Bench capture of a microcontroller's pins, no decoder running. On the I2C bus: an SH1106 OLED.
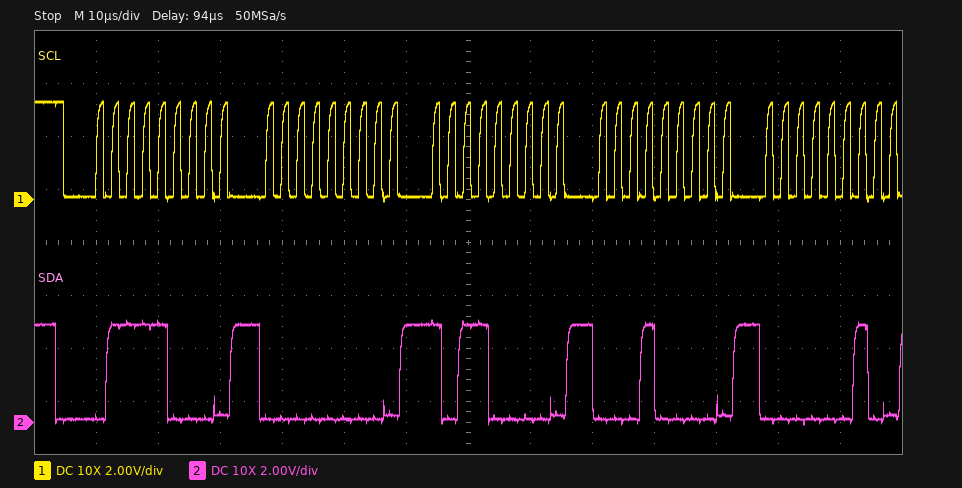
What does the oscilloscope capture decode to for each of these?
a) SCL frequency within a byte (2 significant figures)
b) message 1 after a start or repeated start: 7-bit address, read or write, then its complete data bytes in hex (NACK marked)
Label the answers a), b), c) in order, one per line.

a) 400 kHz
b) 0x3C write: 00 B0 10 02
